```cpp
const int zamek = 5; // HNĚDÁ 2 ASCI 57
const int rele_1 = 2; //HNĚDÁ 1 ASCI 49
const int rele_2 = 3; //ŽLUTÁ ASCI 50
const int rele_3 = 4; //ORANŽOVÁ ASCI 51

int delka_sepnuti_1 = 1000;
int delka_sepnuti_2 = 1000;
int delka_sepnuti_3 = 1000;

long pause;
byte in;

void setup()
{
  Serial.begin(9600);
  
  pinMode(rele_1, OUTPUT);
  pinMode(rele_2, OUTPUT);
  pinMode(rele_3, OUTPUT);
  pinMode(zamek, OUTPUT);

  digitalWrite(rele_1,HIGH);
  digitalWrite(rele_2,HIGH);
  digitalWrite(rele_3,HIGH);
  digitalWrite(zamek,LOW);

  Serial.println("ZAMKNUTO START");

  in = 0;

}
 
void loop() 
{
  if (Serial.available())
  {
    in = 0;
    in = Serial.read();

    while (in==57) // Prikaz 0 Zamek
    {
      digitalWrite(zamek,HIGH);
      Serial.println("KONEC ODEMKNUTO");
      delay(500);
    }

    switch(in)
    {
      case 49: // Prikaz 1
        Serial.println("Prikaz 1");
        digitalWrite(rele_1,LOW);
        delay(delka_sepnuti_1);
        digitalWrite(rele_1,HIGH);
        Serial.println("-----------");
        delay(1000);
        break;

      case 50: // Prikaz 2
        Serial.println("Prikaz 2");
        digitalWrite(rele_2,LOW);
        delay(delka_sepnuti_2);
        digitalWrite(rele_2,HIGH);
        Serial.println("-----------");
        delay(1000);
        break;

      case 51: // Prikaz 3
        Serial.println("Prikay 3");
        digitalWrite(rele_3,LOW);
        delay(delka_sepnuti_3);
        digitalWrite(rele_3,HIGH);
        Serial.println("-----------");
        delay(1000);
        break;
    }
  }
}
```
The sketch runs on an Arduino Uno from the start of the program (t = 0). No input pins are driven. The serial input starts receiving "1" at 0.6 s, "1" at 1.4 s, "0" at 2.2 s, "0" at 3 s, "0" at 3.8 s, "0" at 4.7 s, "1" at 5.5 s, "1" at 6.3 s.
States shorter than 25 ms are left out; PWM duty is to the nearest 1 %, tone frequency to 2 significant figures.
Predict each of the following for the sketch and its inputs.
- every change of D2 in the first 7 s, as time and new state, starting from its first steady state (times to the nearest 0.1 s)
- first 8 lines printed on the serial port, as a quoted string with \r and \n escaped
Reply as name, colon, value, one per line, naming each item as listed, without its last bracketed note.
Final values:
every change of D2 in the first 7 s, as time and new state, starting from its first steady state: 0 s high; 0.6 s low; 1.6 s high; 2.6 s low; 3.6 s high; 5.5 s low; 6.5 s high
first 8 lines printed on the serial port, as a quoted string with \r and \n escaped: "ZAMKNUTO START\r\nPrikaz 1\r\n-----------\r\nPrikaz 1\r\n-----------\r\nPrikaz 1\r\n-----------\r\nPrikaz 1\r\n"
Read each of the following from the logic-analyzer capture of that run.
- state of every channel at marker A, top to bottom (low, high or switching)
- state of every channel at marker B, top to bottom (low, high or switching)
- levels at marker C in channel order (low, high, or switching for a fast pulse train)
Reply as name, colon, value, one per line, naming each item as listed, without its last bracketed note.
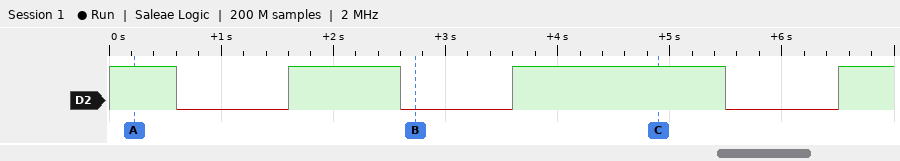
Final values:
state of every channel at marker A, top to bottom: D2 high
state of every channel at marker B, top to bottom: D2 low
levels at marker C in channel order: D2 high
